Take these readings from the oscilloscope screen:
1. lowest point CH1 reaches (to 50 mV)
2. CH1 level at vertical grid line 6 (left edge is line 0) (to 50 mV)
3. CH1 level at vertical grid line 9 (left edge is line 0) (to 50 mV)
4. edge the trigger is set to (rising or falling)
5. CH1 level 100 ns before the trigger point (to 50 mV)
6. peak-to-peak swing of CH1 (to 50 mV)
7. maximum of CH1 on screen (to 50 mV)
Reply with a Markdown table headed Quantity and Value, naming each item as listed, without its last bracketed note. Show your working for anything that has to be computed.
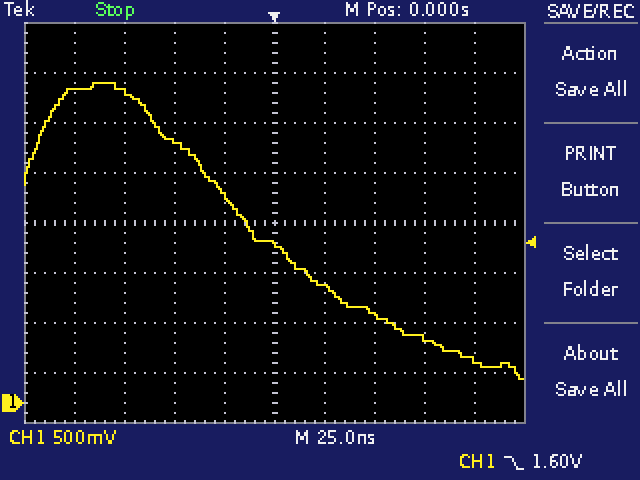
| Quantity | Value |
|---|---|
| lowest point CH1 reaches | 250 mV |
| CH1 level at vertical grid line 6 (left edge is line 0) | 1.15 V |
| CH1 level at vertical grid line 9 (left edge is line 0) | 450 mV |
| edge the trigger is set to | falling |
| CH1 level 100 ns before the trigger point | 3.15 V |
| peak-to-peak swing of CH1 | 3.20 V − (250 mV) = 2.95 V |
| maximum of CH1 on screen | 3.20 V |
